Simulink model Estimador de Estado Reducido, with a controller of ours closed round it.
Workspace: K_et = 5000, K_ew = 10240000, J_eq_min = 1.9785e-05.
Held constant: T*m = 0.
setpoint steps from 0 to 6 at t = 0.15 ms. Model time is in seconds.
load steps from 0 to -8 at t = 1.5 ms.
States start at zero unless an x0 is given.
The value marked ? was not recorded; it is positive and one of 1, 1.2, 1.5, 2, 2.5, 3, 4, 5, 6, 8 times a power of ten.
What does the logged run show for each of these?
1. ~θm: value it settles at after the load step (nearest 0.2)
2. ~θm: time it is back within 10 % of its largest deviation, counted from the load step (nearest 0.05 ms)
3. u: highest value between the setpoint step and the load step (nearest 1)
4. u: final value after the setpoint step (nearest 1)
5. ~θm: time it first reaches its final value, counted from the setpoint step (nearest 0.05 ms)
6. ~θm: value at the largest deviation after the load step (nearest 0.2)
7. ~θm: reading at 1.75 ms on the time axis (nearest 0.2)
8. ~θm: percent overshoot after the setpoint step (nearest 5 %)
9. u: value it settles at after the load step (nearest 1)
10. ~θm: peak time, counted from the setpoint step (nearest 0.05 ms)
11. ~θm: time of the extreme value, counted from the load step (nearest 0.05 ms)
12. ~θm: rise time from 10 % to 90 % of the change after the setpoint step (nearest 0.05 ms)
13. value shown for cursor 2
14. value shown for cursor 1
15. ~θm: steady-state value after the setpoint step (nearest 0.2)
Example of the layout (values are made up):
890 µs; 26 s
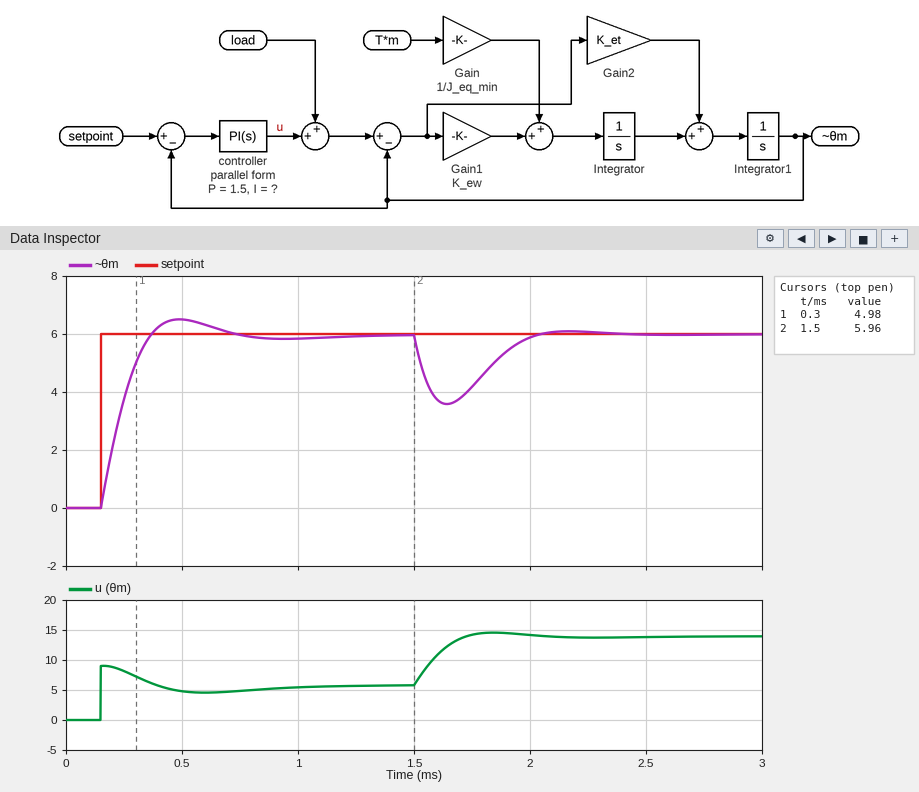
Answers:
6.0; 0.45 ms; 9; 6; 0.20 ms; 3.6; 4.2; 10 %; 14; 0.35 ms; 0.15 ms; 0.15 ms; 5.96; 4.98; 6.0
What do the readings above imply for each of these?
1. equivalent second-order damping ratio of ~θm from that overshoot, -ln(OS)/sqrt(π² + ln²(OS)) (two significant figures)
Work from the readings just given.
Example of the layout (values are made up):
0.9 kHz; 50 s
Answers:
0.59
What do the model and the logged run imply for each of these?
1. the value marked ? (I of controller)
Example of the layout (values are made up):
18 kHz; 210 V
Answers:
12000
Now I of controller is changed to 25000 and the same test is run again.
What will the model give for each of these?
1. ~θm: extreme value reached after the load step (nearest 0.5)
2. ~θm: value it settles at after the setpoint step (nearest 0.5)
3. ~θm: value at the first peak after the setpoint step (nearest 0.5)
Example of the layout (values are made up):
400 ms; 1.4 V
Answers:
4.0; 6.0; 7.5
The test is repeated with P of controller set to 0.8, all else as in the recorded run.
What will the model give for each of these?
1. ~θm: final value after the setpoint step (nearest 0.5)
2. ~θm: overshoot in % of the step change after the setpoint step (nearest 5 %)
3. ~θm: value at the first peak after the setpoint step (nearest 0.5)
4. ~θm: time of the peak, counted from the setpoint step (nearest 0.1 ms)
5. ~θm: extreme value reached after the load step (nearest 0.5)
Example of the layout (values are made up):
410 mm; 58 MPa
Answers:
6.0; 20 %; 7.0; 0.4 ms; 3.0
